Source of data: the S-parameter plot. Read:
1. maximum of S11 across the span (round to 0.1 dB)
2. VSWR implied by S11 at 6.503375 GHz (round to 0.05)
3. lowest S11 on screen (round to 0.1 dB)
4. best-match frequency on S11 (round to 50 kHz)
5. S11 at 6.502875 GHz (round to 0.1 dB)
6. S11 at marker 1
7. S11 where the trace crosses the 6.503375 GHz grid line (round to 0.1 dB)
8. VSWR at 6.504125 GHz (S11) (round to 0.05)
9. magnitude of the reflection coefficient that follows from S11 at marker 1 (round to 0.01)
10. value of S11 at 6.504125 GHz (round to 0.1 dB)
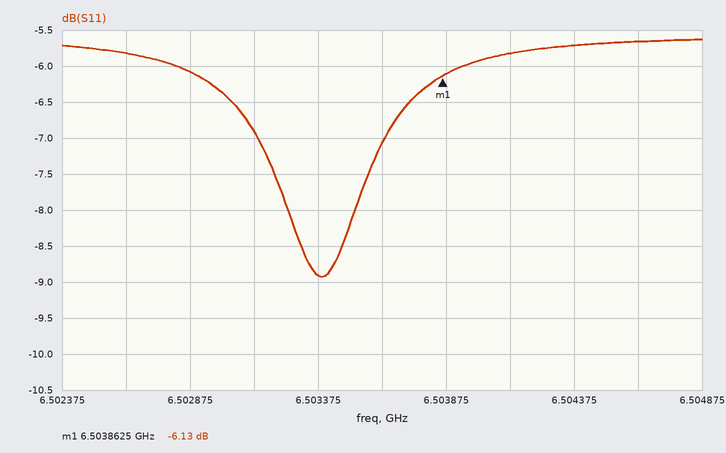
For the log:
-5.6 dB
2.10
-8.9 dB
6.50340 GHz
-6.1 dB
-6.13 dB
-8.9 dB
3.10
0.49
-5.8 dB
